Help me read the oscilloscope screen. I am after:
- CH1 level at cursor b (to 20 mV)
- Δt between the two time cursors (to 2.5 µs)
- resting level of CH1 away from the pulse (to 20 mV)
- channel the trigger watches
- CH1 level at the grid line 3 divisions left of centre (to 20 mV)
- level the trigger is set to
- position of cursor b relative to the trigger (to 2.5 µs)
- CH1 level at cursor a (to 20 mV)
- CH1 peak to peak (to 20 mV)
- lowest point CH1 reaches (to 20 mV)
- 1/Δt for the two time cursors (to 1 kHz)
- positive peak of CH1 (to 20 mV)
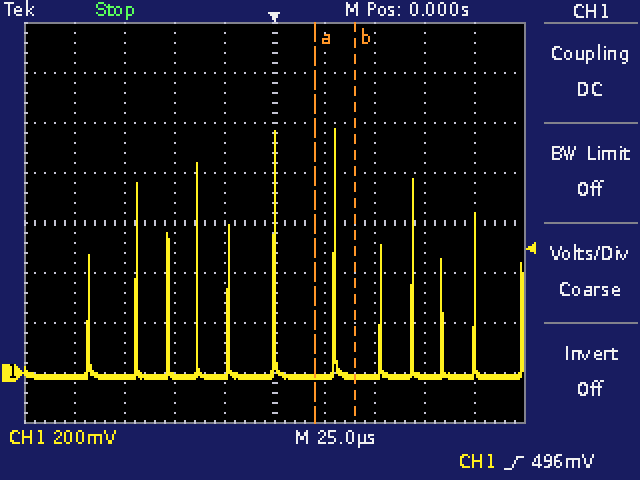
-20 mV
20.0 µs
-20 mV
CH1
-20 mV
496 mV
+40.0 µs
-20 mV
1.00 V
-20 mV
50 kHz
980 mV
